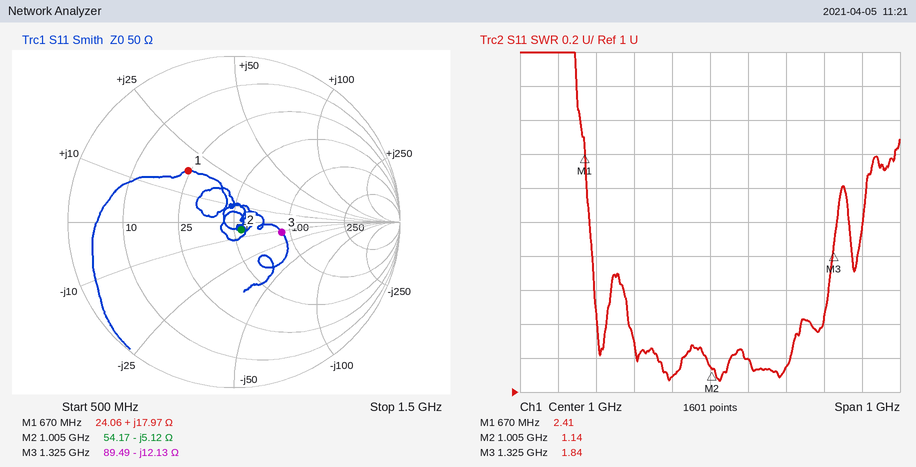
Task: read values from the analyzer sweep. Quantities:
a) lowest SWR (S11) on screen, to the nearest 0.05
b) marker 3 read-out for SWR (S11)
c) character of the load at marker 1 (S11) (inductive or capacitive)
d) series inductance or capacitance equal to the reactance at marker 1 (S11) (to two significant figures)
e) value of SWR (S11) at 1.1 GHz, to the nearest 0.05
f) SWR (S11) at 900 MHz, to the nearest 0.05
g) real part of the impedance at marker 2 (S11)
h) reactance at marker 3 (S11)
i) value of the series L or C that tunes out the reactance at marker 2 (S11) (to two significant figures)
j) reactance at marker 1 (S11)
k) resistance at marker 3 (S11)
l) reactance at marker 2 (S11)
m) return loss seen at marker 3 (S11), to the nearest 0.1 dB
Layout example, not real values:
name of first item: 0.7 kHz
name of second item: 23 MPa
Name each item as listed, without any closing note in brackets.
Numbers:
lowest SWR (S11) on screen, to the nearest 0.05: 1.05
marker 3 read-out for SWR: 1.84
character of the load at marker 1 (S11): inductive
series inductance or capacitance equal to the reactance at marker 1 (S11): 4.3 nH
value of SWR (S11) at 1.1 GHz, to the nearest 0.05: 1.20
SWR (S11) at 900 MHz, to the nearest 0.05: 1.10
real part of the impedance at marker 2: 54.17 Ω
reactance at marker 3: -12.13 Ω
value of the series L or C that tunes out the reactance at marker 2 (S11): 810 pH
reactance at marker 1: +17.97 Ω
resistance at marker 3: 89.49 Ω
reactance at marker 2: -5.12 Ω
return loss seen at marker 3 (S11), to the nearest 0.1 dB: 10.6 dB
